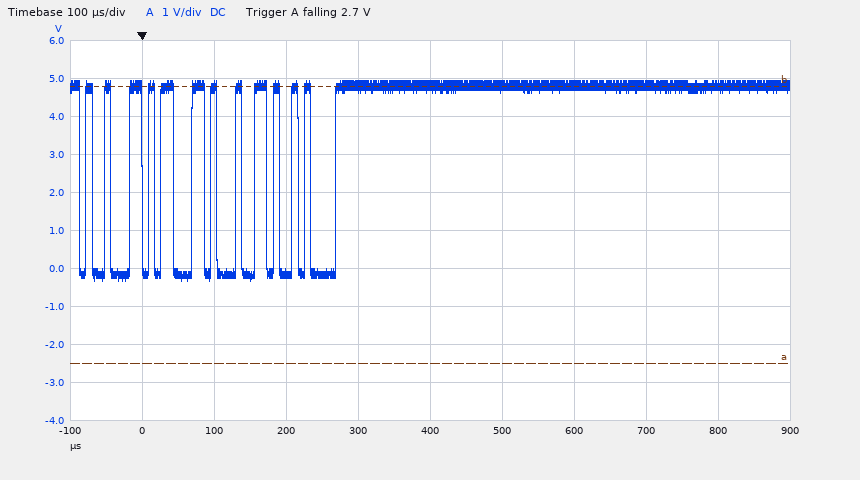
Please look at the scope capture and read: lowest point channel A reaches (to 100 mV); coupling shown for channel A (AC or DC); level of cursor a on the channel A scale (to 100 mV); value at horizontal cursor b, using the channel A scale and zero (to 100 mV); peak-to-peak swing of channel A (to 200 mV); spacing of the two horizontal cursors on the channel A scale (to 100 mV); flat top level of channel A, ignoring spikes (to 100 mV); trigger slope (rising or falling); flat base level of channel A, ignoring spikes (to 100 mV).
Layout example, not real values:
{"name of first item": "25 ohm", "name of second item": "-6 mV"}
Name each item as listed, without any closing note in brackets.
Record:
{"lowest point channel A reaches": "-300 mV", "coupling shown for channel A": "DC", "level of cursor a on the channel A scale": "-2.5 V", "value at horizontal cursor b, using the channel A scale and zero": "4.8 V", "peak-to-peak swing of channel A": "5.2 V", "spacing of the two horizontal cursors on the channel A scale": "7.3 V", "flat top level of channel A, ignoring spikes": "4.8 V", "trigger slope": "falling", "flat base level of channel A, ignoring spikes": "-200 mV"}
